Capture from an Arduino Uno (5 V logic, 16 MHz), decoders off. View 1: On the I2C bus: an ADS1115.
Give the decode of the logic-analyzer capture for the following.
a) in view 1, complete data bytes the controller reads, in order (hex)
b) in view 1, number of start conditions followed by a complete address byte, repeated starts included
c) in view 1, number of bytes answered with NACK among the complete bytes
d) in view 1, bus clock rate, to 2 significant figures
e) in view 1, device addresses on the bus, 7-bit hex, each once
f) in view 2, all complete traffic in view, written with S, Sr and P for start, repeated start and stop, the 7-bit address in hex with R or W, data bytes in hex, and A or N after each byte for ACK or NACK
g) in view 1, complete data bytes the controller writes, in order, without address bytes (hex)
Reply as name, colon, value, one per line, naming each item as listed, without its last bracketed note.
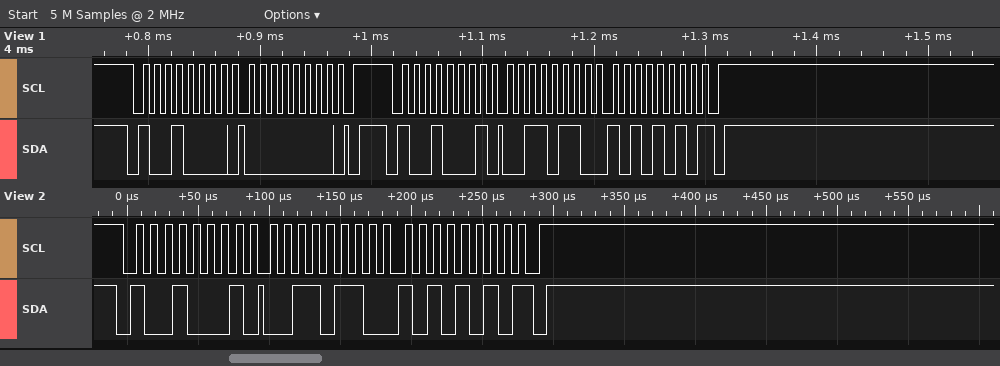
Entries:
in view 1, complete data bytes the controller reads, in order: 36 AA
in view 1, number of start conditions followed by a complete address byte, repeated starts included: 2
in view 1, number of bytes answered with NACK among the complete bytes: 1
in view 1, bus clock rate, to 2 significant figures: 100 kHz
in view 1, device addresses on the bus, 7-bit hex, each once: 0x48
in view 2, all complete traffic in view, written with S, Sr and P for start, repeated start and stop, the 7-bit address in hex with R or W, data bytes in hex, and A or N after each byte for ACK or NACK: S 48R A 36 A AA N P
in view 1, complete data bytes the controller writes, in order, without address bytes: 00
